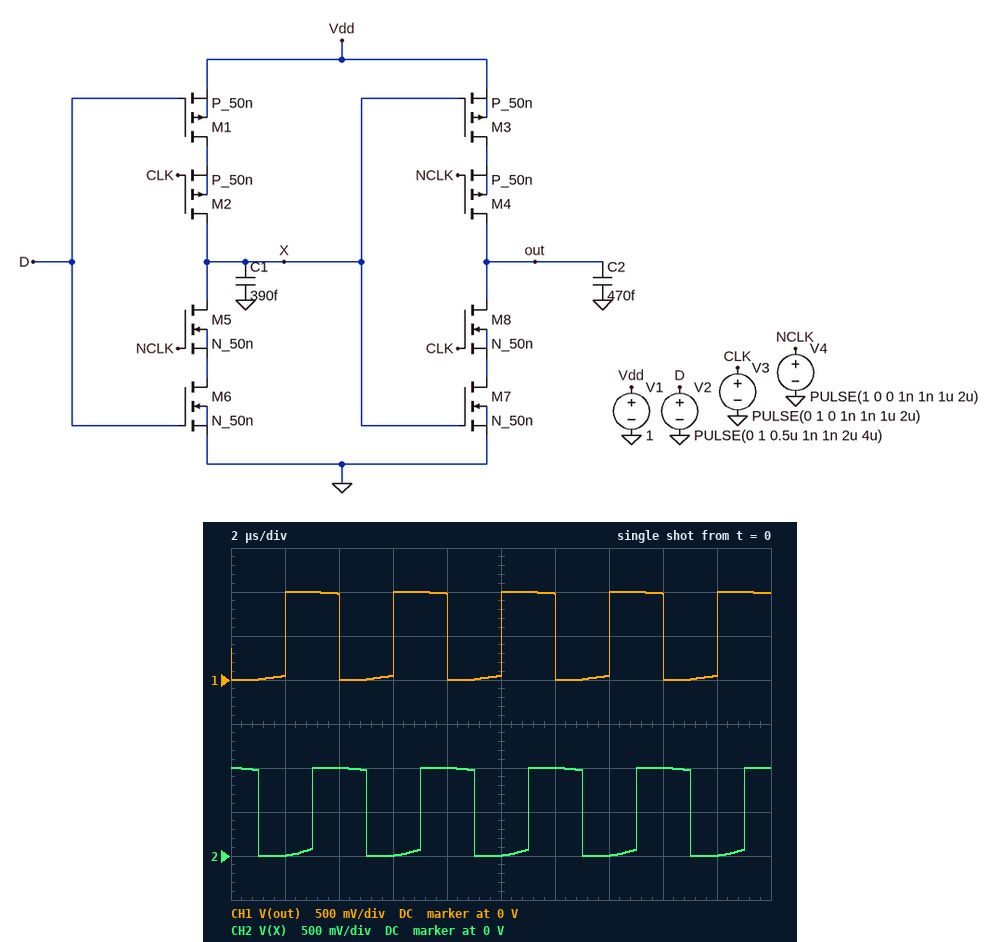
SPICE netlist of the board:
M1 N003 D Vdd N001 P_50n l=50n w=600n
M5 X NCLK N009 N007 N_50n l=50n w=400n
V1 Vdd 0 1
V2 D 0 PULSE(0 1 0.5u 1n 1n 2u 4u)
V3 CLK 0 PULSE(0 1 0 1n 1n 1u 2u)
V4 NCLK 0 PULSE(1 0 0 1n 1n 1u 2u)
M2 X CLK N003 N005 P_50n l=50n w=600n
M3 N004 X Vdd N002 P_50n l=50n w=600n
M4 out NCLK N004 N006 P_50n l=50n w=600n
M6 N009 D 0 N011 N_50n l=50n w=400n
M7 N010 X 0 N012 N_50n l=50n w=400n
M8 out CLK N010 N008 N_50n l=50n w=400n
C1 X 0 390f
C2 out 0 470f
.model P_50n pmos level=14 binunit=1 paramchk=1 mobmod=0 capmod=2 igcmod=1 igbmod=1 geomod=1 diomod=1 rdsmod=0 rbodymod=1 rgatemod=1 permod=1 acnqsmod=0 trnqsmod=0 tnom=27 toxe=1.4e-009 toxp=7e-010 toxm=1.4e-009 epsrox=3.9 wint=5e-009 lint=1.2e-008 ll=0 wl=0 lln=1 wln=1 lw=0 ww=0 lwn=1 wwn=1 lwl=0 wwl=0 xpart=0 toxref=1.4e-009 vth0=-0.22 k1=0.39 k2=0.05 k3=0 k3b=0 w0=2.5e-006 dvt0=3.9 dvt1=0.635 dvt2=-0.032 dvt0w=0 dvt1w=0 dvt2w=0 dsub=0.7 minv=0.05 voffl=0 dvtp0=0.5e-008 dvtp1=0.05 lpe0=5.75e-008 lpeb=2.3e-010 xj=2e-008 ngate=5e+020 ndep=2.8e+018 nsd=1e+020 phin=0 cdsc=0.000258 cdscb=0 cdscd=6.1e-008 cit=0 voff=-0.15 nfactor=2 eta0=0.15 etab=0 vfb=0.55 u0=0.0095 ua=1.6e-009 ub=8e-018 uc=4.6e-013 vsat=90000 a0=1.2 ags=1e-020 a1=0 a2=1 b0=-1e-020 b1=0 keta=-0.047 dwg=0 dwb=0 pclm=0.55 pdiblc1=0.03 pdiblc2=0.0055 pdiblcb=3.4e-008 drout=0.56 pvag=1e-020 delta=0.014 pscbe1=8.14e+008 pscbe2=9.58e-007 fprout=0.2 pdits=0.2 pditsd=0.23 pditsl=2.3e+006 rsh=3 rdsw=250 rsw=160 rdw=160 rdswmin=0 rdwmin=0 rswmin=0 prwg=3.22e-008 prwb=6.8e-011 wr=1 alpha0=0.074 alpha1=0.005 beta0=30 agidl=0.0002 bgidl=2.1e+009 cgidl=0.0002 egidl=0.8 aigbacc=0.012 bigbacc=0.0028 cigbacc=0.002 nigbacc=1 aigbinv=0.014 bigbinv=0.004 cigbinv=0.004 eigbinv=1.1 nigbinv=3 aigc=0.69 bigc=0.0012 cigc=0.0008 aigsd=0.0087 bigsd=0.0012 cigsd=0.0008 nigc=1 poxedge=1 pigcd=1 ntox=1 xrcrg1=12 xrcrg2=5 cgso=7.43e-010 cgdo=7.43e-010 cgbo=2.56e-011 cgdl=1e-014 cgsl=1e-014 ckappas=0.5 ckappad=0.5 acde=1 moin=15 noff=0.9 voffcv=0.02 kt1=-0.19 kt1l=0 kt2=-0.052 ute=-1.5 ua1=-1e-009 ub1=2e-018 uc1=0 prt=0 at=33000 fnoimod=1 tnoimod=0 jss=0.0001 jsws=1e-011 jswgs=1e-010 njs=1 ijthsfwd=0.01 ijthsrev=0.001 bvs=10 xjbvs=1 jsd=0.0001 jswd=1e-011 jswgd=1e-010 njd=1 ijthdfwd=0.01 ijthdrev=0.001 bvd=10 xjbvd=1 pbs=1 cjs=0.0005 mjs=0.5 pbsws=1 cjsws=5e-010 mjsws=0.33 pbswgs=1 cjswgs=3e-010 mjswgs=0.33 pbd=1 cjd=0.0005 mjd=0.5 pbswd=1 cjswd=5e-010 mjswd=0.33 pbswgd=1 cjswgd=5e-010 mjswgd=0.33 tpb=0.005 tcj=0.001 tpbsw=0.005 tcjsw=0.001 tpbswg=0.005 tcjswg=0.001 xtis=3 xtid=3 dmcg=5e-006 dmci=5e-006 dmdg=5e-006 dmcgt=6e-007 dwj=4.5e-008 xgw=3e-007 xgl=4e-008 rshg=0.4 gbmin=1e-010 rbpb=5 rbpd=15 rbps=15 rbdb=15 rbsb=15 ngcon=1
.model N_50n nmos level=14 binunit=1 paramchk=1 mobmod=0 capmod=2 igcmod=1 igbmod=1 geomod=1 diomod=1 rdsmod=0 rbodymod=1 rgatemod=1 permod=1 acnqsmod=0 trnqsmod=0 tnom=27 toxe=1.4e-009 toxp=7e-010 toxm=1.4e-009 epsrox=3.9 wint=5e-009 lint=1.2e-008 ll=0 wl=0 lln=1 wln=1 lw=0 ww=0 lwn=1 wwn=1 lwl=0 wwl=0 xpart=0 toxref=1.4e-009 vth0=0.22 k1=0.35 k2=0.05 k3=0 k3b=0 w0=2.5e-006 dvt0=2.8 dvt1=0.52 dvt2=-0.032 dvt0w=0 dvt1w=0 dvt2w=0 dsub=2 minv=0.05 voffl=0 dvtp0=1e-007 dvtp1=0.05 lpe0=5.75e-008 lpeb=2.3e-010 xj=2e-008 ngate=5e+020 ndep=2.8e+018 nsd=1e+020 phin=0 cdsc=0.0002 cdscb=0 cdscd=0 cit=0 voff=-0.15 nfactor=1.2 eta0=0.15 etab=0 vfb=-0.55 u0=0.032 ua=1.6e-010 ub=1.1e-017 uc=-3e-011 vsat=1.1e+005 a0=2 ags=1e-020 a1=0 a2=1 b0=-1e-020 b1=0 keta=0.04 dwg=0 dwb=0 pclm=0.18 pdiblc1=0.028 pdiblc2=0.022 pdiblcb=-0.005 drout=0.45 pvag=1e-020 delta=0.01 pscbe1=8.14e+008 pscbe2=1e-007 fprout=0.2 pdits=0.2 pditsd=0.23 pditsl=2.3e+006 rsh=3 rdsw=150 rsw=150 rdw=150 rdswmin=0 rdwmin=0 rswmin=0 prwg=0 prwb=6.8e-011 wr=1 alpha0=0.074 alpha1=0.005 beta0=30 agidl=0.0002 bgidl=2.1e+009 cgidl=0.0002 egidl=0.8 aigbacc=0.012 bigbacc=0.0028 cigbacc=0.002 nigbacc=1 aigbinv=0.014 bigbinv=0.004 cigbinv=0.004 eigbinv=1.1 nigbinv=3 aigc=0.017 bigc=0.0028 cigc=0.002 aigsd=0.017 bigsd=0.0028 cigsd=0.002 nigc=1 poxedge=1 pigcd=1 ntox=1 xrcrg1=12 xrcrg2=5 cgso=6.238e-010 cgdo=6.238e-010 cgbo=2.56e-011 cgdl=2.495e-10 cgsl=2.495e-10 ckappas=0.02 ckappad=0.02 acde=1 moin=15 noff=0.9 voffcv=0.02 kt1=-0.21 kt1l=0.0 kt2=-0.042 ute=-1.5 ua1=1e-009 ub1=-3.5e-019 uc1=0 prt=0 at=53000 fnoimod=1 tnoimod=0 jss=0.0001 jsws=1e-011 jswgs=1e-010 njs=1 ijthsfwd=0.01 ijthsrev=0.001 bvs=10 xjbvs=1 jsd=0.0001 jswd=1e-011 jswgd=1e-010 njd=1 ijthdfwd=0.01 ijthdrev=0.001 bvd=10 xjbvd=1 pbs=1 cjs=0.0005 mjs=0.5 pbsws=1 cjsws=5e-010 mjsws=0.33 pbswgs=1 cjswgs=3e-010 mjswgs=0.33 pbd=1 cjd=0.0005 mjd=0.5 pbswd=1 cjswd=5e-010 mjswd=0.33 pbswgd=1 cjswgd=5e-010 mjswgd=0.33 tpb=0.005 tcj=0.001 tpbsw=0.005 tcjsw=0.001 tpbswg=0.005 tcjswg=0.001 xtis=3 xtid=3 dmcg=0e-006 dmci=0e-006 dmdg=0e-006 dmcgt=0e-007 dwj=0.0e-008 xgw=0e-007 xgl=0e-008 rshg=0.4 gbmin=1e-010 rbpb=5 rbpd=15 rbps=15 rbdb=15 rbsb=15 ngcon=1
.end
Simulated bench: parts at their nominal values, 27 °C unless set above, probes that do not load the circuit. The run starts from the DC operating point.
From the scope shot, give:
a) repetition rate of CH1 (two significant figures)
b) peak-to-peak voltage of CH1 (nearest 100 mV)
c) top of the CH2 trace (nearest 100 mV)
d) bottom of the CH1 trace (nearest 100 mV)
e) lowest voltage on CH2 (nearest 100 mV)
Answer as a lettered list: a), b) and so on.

a) 250 kHz
b) 1.0 V
c) 1.0 V
d) 0 V
e) 0 V
